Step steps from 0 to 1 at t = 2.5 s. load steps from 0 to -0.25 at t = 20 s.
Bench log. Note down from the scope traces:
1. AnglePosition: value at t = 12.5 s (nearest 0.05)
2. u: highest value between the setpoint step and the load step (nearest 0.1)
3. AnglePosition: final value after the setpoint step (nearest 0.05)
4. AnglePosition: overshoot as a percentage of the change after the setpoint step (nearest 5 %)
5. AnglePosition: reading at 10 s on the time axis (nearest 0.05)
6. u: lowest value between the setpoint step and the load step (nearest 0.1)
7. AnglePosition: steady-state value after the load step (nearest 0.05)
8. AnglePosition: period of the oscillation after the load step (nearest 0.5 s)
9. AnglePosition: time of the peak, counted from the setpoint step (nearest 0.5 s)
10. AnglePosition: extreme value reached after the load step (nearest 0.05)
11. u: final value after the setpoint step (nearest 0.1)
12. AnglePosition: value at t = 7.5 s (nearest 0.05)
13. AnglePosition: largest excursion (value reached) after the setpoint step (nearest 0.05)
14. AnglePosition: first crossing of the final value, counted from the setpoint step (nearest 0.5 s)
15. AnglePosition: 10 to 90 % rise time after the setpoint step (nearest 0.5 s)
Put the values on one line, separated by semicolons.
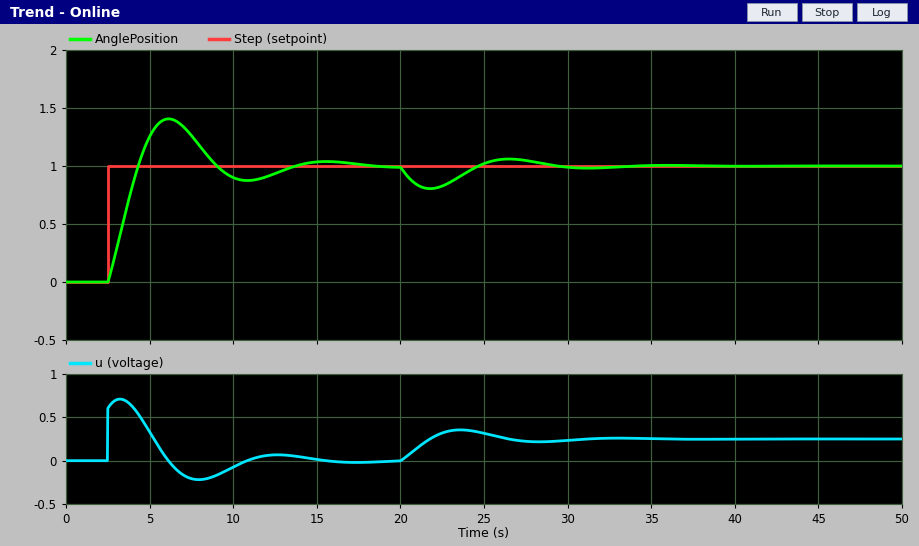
0.95; 0.7; 1.00; 40 %; 0.90; -0.2; 1.00; 9.5 s; 3.5 s; 0.80; 0.0; 1.25; 1.40; 2.0 s; 1.5 s
